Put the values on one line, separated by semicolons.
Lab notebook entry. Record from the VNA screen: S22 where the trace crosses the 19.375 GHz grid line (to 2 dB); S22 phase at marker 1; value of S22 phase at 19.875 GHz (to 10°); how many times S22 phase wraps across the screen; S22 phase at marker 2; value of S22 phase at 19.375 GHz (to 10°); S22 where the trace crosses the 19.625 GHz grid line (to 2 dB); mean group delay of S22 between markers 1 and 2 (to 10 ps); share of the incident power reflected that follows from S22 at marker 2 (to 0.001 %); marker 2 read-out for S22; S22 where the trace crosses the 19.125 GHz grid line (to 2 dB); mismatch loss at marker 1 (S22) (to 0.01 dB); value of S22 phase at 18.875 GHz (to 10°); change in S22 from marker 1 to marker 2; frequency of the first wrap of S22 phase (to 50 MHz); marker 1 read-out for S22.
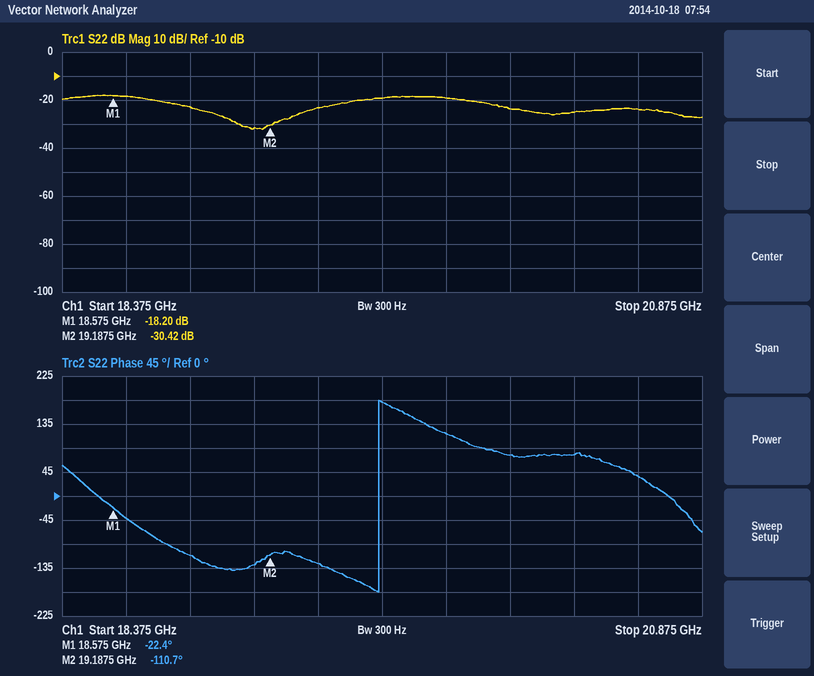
-24 dB; -22.4°; 120°; 1; -110.7°; -130°; -20 dB; 400 ps; 0.091 %; -30.42 dB; -32 dB; 0.07 dB; -110°; -12.22 dB; 19.60 GHz; -18.20 dB
